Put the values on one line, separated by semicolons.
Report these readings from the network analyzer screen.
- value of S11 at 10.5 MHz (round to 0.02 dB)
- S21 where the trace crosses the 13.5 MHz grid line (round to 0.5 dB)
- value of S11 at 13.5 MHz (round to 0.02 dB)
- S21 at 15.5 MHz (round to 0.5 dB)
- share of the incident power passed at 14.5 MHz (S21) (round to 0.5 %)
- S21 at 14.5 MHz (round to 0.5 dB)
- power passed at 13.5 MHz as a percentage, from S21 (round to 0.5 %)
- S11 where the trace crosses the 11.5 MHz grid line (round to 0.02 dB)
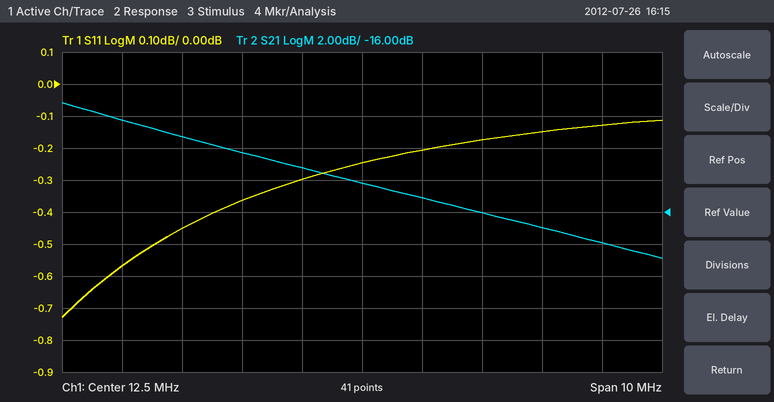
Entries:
-0.36 dB; -15.0 dB; -0.20 dB; -17.0 dB; 2.5 %; -16.0 dB; 3.0 %; -0.30 dB
